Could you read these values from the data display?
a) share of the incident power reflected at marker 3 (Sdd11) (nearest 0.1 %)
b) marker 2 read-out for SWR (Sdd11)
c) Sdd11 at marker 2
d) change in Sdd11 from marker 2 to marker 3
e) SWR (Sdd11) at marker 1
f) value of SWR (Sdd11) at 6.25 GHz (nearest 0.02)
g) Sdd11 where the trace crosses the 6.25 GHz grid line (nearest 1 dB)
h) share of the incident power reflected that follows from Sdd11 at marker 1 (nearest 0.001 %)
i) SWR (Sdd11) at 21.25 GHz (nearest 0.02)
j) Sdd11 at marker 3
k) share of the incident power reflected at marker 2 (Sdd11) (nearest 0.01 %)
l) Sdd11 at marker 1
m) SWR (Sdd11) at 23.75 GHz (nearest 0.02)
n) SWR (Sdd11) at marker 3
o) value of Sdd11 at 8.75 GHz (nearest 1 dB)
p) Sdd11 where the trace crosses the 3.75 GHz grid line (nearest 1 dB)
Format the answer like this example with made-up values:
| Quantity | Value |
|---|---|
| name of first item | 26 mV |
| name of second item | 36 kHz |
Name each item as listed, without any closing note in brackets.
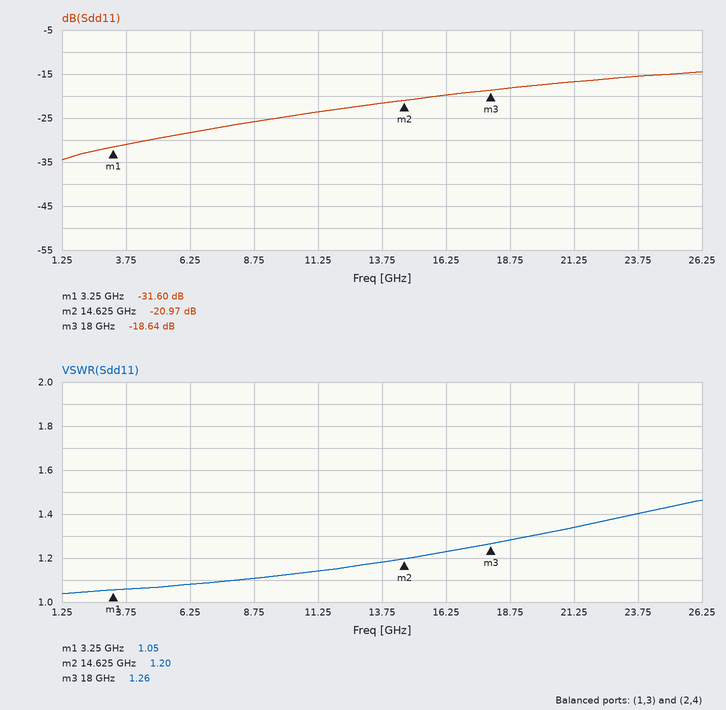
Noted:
| Quantity | Value |
|---|---|
| share of the incident power reflected at marker 3 (Sdd11) | 1.4 % |
| marker 2 read-out for SWR | 1.20 |
| Sdd11 at marker 2 | -20.97 dB |
| change in Sdd11 from marker 2 to marker 3 | 2.33 dB |
| SWR (Sdd11) at marker 1 | 1.05 |
| value of SWR (Sdd11) at 6.25 GHz | 1.08 |
| Sdd11 where the trace crosses the 6.25 GHz grid line | -28 dB |
| share of the incident power reflected that follows from Sdd11 at marker 1 | 0.069 % |
| SWR (Sdd11) at 21.25 GHz | 1.34 |
| Sdd11 at marker 3 | -18.64 dB |
| share of the incident power reflected at marker 2 (Sdd11) | 0.80 % |
| Sdd11 at marker 1 | -31.60 dB |
| SWR (Sdd11) at 23.75 GHz | 1.40 |
| SWR (Sdd11) at marker 3 | 1.26 |
| value of Sdd11 at 8.75 GHz | -26 dB |
| Sdd11 where the trace crosses the 3.75 GHz grid line | -31 dB |
